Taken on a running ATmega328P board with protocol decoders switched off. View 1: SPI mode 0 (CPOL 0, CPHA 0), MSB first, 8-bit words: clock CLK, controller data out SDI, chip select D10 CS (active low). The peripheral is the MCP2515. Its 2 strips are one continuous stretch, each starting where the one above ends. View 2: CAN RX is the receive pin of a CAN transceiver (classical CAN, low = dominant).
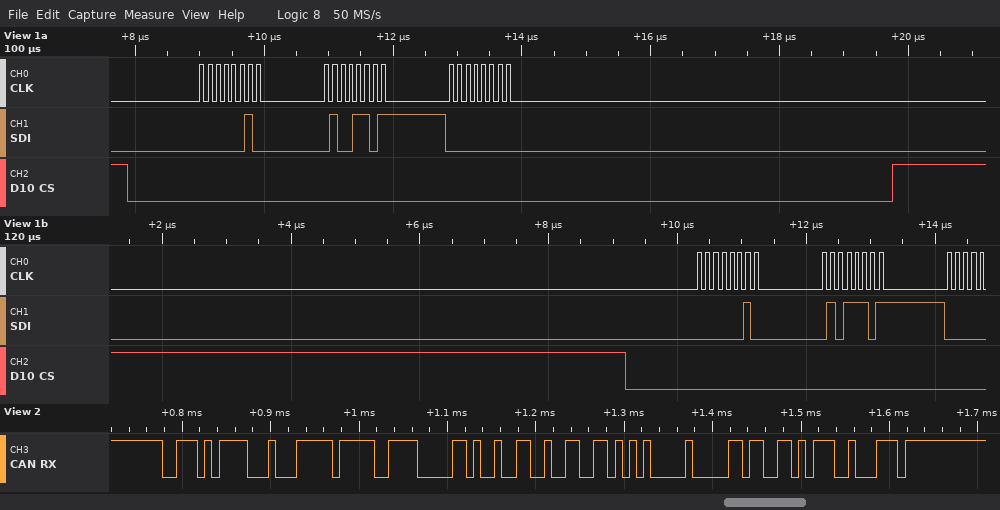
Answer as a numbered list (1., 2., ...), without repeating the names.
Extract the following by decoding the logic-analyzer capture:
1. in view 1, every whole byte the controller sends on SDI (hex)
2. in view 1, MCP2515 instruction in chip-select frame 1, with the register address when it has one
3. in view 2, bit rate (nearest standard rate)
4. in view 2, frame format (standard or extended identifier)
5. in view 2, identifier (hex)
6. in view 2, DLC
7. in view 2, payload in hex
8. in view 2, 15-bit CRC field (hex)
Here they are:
1. 02 4D 00 02 5D
2. WRITE 0x4D
3. 125 kbit/s
4. standard
5. 0x3AF
6. 8
7. FF DE 0A 4C 99 AA 00 59
8. 0x5723
